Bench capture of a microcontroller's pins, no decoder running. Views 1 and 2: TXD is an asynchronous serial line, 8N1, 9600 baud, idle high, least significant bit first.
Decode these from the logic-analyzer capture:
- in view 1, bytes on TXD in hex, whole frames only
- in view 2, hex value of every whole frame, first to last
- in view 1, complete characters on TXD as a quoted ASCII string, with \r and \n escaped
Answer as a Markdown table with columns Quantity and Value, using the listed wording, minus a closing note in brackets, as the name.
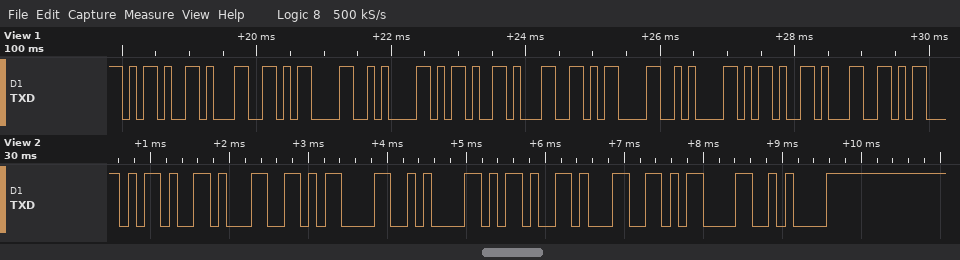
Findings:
| Quantity | Value |
|---|---|
| in view 1, bytes on TXD in hex, whole frames only | 0x2D 0x31 0x0D 0x0A 0x2D 0x31 0x0D 0x0A 0x2D 0x31 |
| in view 2, hex value of every whole frame, first to last | 2D 31 0D 0A 2D 31 0D 0A |
| in view 1, complete characters on TXD as a quoted ASCII string, with \r and \n escaped | "-1\r\n-1\r\n-1" |
